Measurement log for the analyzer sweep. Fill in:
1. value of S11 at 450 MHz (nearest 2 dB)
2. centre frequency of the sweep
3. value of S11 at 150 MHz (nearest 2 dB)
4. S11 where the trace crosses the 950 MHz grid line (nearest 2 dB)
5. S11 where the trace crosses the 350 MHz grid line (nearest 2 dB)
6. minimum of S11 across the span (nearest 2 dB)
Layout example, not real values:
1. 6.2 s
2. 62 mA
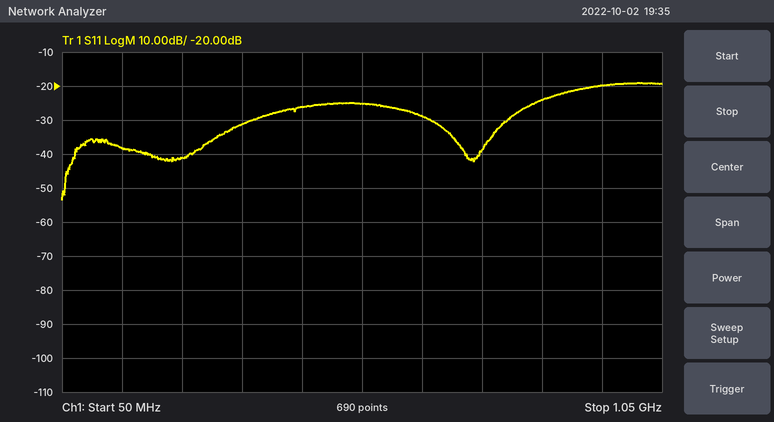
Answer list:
1. -26 dB
2. 550 MHz
3. -38 dB
4. -20 dB
5. -32 dB
6. -54 dB
